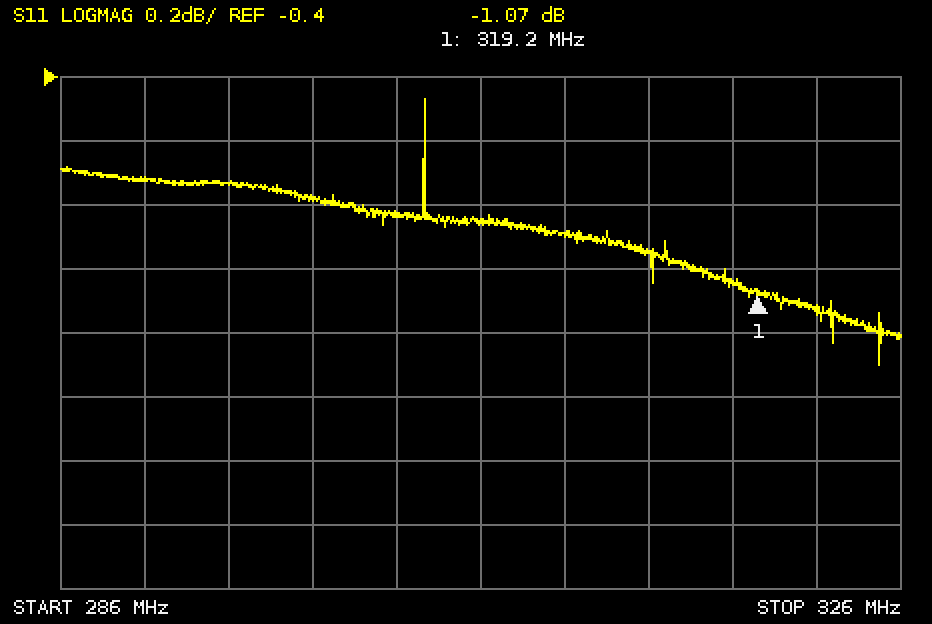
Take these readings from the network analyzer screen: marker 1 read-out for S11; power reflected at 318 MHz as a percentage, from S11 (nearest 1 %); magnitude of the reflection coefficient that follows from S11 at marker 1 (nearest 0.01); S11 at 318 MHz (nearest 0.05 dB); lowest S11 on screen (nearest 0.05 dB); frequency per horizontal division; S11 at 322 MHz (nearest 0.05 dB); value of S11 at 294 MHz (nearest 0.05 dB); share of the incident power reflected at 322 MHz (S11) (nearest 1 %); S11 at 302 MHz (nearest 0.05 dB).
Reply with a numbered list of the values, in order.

1. -1.07 dB
2. 79 %
3. 0.88
4. -1.05 dB
5. -1.30 dB
6. 4 MHz
7. -1.15 dB
8. -0.75 dB
9. 77 %
10. -0.85 dB
